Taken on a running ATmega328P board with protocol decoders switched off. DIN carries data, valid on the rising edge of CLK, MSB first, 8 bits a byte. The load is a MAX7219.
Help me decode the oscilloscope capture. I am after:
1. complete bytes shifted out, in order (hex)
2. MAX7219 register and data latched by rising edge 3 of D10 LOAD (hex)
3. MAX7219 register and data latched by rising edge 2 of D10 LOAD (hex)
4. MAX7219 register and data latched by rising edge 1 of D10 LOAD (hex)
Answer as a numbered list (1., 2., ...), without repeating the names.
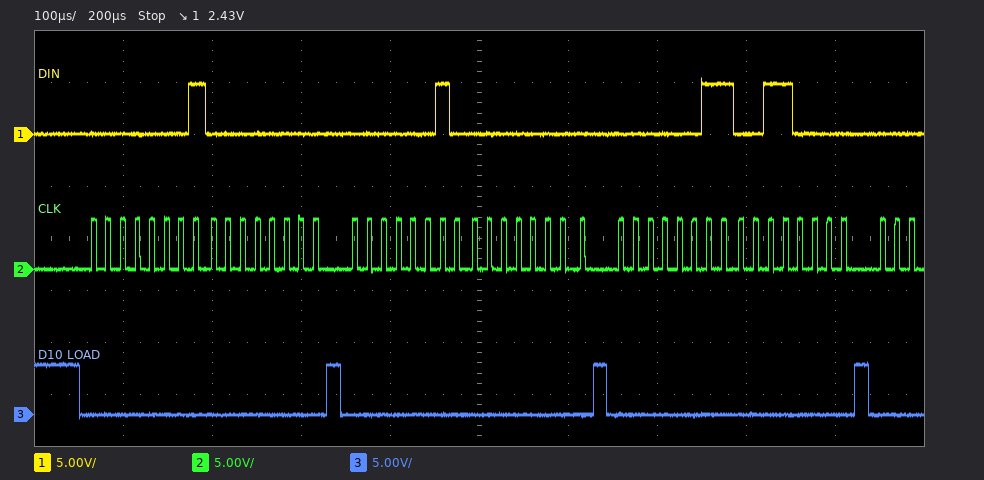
1. 01 00 02 00 03 30
2. register 0x3, data 0x30
3. register 0x2, data 0x00
4. register 0x1, data 0x00
